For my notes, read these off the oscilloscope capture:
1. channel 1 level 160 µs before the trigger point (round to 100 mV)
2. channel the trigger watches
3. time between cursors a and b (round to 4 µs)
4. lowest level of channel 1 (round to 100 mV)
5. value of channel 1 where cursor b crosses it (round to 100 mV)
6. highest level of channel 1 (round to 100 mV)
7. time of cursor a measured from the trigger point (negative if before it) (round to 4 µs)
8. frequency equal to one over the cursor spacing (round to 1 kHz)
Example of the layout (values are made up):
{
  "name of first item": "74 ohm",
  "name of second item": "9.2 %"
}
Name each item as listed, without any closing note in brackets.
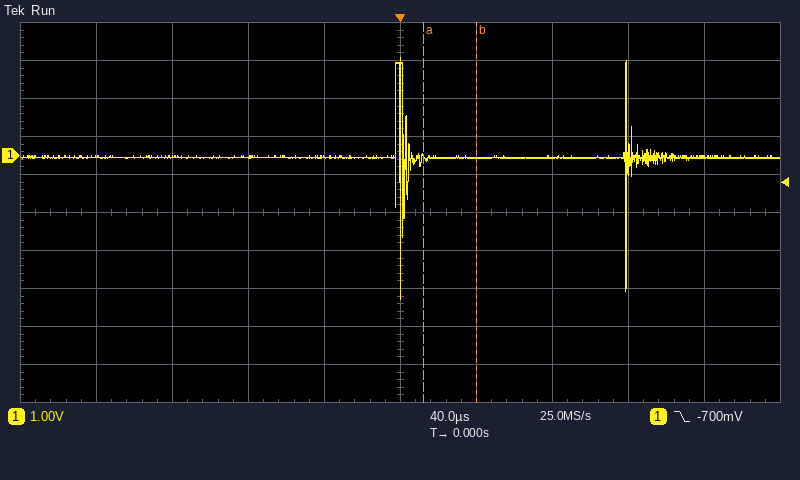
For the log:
{
  "channel 1 level 160 µs before the trigger point": "0.0 V",
  "channel the trigger watches": "channel 1",
  "time between cursors a and b": "28 µs",
  "lowest level of channel 1": "-3.8 V",
  "value of channel 1 where cursor b crosses it": "-100 mV",
  "highest level of channel 1": "2.6 V",
  "time of cursor a measured from the trigger point (negative if before it)": "+12 µs",
  "frequency equal to one over the cursor spacing": "36 kHz"
}
